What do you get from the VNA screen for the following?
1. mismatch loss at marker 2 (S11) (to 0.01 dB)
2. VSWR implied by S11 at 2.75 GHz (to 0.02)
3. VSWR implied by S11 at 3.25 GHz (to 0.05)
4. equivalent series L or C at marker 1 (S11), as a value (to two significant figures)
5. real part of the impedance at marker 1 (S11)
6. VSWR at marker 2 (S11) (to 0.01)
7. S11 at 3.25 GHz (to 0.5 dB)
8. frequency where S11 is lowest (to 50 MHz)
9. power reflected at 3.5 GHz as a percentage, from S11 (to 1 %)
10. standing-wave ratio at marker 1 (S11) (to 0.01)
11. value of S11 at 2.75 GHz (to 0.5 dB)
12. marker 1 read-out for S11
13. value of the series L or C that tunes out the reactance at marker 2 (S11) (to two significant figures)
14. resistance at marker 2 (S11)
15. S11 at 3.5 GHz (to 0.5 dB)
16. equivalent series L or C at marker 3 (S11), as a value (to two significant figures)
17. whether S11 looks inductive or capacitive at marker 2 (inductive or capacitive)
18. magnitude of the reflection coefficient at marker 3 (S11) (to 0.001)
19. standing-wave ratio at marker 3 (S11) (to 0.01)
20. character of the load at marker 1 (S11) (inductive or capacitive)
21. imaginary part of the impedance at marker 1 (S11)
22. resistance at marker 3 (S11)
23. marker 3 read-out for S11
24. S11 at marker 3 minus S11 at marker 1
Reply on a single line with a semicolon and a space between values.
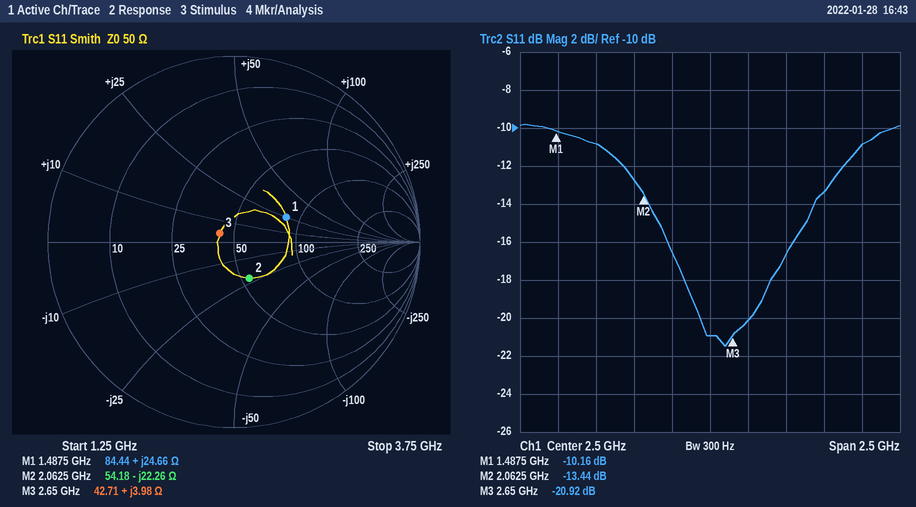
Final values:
0.20 dB; 1.22; 1.55; 2.6 nH; 84.44 Ω; 1.54; -13.5 dB; 2.60 GHz; 8 %; 1.90; -20.0 dB; -10.16 dB; 1.7 nH; 54.18 Ω; -11.0 dB; 240 pH; capacitive; 0.090; 1.20; inductive; +24.66 Ω; 42.71 Ω; -20.92 dB; -10.76 dB
